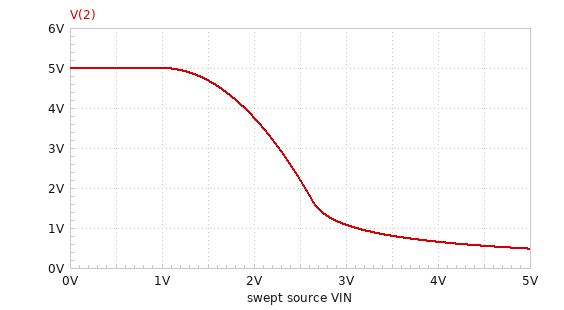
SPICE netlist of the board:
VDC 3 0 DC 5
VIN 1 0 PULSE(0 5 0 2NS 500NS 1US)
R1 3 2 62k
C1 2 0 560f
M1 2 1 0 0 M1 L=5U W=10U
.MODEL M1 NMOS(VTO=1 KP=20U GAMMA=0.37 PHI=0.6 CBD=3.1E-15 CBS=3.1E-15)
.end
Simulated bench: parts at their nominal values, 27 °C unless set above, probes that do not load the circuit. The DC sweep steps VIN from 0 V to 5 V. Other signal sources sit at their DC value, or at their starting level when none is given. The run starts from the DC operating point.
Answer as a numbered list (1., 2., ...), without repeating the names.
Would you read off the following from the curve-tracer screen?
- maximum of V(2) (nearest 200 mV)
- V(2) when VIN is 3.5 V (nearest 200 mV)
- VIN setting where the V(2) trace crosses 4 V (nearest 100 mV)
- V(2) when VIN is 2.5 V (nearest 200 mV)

1. 5.0 V
2. 800 mV
3. 1.9 V
4. 2.2 V
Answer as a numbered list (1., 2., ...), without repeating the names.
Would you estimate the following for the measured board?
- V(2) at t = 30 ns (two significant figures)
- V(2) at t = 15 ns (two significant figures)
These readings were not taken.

1. 490 mV
2. 720 mV
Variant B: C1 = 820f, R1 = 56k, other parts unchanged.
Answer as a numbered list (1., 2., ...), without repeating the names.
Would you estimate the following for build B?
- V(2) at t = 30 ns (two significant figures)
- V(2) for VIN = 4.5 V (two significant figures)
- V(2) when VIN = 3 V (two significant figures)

1. 580 mV
2. 610 mV
3. 1.2 V
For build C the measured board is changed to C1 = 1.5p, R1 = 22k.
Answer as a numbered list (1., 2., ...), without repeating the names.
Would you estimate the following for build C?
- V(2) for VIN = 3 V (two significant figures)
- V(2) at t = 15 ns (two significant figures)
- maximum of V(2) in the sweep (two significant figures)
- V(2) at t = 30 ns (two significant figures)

1. 3.2 V
2. 2.7 V
3. 5.0 V
4. 1.6 V
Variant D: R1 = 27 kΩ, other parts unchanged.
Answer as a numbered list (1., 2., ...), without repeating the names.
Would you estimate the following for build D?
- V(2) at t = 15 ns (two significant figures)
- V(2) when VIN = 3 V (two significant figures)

1. 1.2 V
2. 2.8 V
